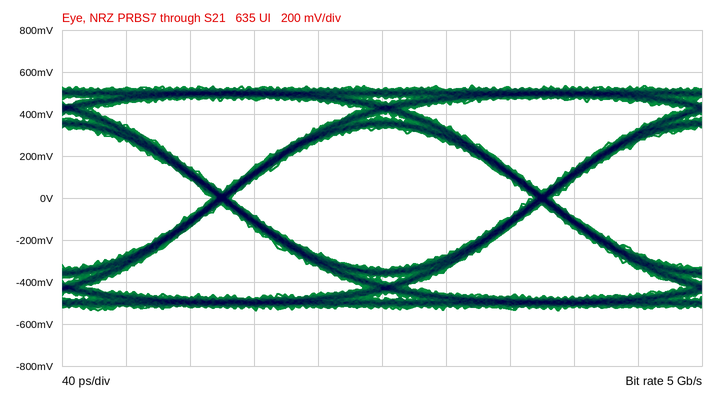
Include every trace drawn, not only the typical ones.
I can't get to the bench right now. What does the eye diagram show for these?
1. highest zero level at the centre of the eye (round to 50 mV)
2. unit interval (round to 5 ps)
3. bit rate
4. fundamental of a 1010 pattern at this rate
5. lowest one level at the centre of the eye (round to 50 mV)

-350 mV
200 ps
5 Gb/s
2.5 GHz
350 mV
